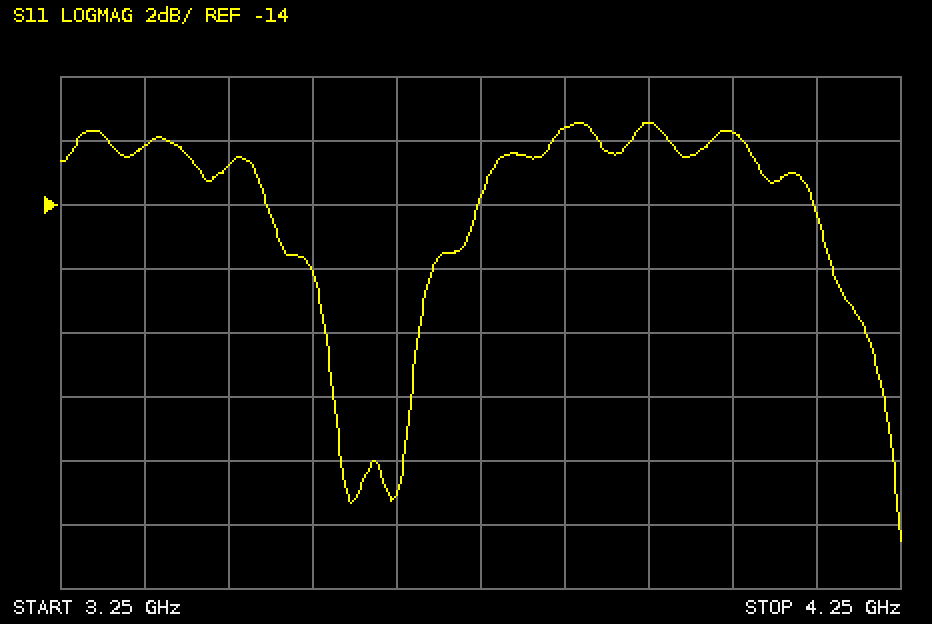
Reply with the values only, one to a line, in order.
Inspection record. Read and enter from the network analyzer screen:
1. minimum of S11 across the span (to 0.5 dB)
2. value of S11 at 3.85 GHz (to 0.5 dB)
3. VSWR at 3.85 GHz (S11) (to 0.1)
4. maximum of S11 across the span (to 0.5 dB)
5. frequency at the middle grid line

-24.5 dB
-11.5 dB
1.7
-11.5 dB
3.75 GHz
